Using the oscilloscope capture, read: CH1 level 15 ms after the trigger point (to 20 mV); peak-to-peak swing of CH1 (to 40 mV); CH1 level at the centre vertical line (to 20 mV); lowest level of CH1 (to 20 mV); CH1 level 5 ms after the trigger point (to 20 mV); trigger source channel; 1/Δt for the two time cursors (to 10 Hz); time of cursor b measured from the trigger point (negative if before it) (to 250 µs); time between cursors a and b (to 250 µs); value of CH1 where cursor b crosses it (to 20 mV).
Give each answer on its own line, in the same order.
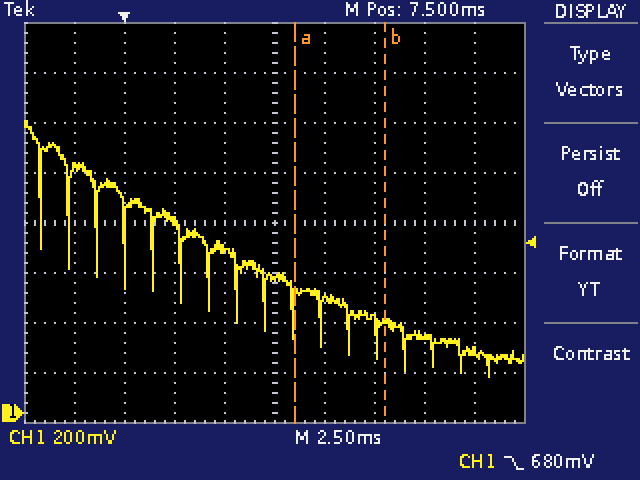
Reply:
300 mV
1.04 V
540 mV
140 mV
660 mV
CH1
220 Hz
+13.00 ms
4.50 ms
360 mV
